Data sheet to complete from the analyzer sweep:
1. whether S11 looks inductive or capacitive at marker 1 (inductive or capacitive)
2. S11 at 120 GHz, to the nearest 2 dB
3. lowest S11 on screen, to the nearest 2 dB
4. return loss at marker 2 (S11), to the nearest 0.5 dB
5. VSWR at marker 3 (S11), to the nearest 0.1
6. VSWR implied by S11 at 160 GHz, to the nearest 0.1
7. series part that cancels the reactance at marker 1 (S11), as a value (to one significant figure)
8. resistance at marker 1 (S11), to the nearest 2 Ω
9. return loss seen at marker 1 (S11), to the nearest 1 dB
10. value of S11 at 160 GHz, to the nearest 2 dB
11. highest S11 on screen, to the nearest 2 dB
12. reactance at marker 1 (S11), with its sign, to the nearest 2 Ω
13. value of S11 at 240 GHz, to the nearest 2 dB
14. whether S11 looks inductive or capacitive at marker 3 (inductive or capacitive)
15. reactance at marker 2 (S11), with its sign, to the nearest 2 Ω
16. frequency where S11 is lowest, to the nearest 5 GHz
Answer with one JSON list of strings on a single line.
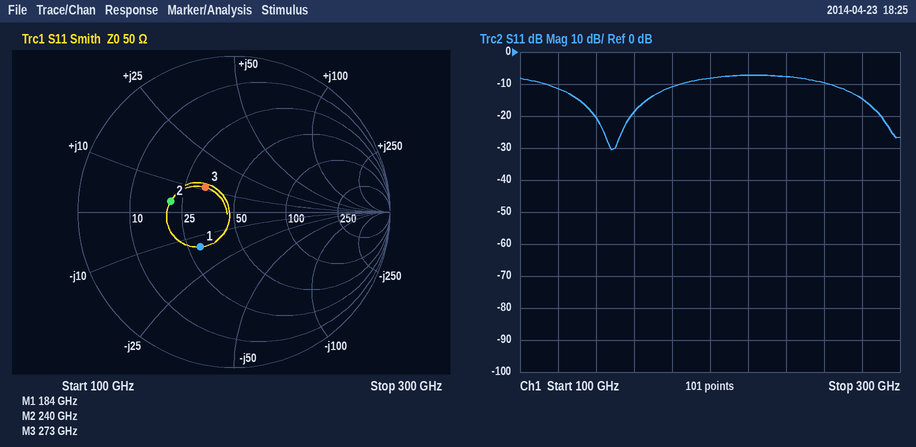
["capacitive", "-12 dB", "-30 dB", "7.5 dB", "1.6", "1.3", "10 pH", "30 Ω", "10 dB", "-18 dB", "-8 dB", "-14 Ω", "-8 dB", "inductive", "+4 Ω", "150 GHz"]
